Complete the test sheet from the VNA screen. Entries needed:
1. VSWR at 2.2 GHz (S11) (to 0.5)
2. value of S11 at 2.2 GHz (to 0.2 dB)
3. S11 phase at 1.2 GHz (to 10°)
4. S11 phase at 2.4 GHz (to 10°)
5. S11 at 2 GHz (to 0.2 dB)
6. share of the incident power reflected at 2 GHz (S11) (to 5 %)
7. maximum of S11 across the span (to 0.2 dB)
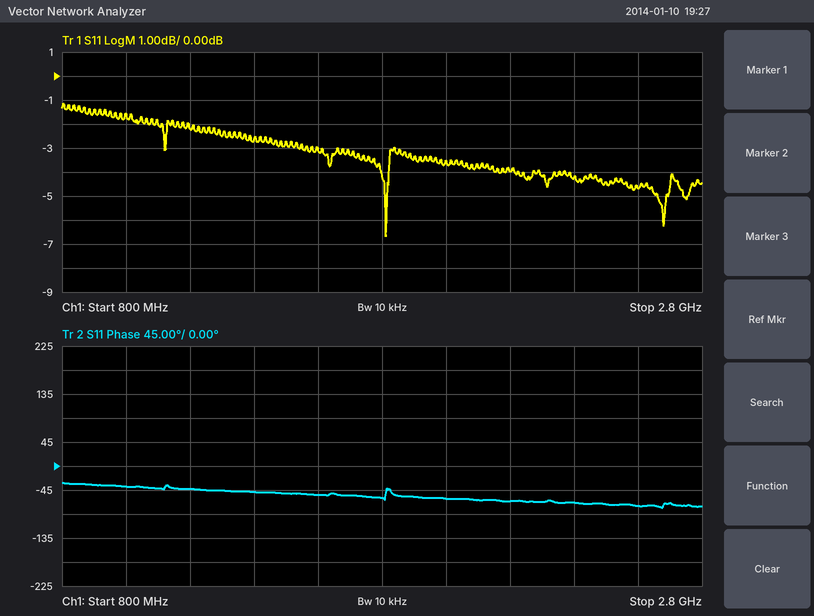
4.5
-4.0 dB
-40°
-70°
-3.6 dB
45 %
-1.2 dB
